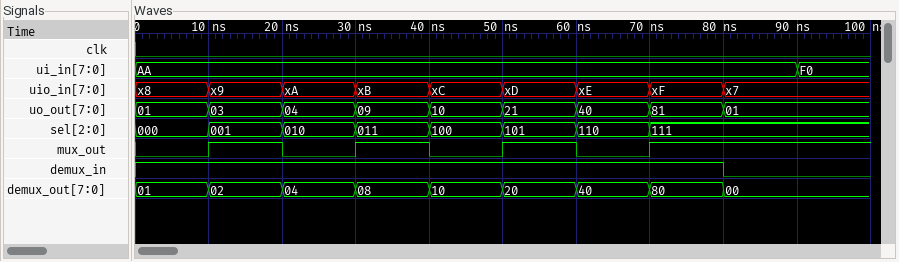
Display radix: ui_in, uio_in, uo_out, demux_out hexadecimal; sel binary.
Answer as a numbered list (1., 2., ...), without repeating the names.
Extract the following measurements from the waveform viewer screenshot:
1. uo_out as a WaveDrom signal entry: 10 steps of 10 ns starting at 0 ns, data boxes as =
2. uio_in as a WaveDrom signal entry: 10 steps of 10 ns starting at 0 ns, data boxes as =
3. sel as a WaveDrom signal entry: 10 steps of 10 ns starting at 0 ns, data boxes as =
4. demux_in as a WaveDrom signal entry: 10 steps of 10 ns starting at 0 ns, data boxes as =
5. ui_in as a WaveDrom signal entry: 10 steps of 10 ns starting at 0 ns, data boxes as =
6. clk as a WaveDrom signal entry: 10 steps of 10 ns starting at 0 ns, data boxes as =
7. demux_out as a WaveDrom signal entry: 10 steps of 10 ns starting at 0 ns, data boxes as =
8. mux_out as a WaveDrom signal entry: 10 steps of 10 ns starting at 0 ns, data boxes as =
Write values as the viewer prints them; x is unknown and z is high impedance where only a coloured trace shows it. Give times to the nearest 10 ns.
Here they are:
1. {name: 'uo_out', wave: '=========.', data: '01 03 04 09 10 21 40 81 01'}
2. {name: 'uio_in', wave: '=========.', data: 'x8 x9 xA xB xC xD xE xF x7'}
3. {name: 'sel', wave: '========..', data: '000 001 010 011 100 101 110 111'}
4. {name: 'demux_in', wave: '1.......0.'}
5. {name: 'ui_in', wave: '=........=', data: 'AA F0'}
6. {name: 'clk', wave: '0.........'}
7. {name: 'demux_out', wave: '=========.', data: '01 02 04 08 10 20 40 80 00'}
8. {name: 'mux_out', wave: '01010101..'}
